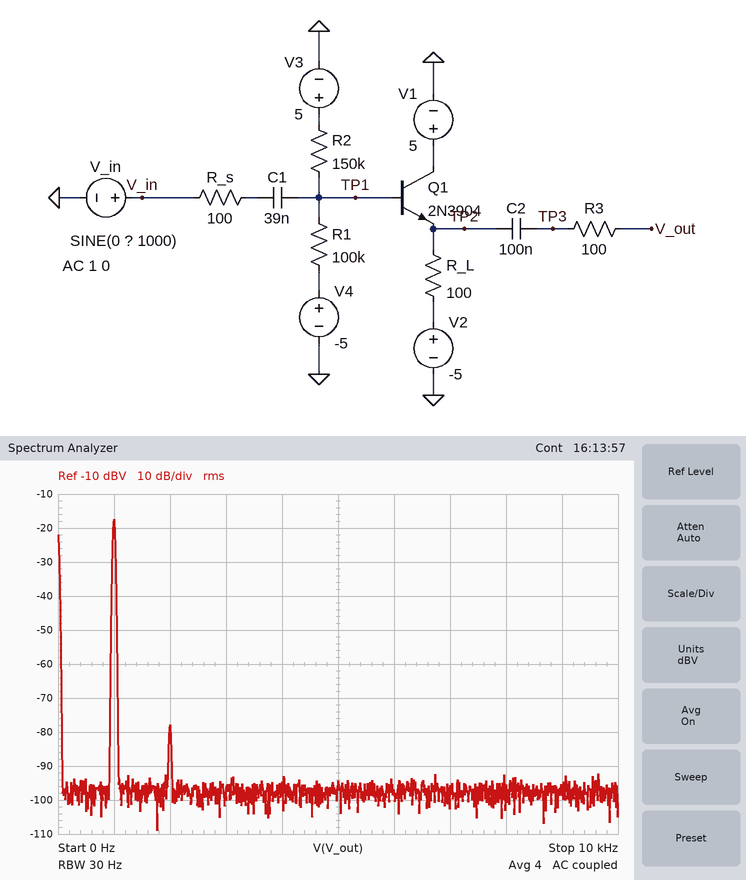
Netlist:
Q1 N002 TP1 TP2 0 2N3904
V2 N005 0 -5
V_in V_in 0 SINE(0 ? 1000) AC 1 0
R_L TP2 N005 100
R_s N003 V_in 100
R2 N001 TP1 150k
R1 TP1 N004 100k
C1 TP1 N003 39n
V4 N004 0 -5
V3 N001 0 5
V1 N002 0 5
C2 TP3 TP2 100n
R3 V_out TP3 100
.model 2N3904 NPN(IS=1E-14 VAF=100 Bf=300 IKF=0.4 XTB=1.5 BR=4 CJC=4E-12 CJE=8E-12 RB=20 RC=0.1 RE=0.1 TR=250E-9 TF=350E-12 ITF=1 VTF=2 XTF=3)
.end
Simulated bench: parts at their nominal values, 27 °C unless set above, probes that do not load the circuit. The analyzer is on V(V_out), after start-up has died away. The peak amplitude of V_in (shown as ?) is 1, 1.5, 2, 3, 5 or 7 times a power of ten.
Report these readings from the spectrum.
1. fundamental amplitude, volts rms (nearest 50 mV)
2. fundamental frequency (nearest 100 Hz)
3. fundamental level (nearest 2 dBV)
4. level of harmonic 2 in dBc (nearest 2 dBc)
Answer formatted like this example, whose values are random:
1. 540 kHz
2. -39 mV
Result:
1. 150 mV
2. 1.0 kHz
3. -18 dBV
4. -60 dBc
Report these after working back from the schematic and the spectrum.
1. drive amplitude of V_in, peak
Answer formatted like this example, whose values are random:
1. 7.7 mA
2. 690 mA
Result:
1. 200 mV
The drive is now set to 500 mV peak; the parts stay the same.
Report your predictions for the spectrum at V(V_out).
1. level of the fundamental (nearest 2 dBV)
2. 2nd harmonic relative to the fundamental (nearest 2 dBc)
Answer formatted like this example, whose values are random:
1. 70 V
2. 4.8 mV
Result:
1. -10 dBV
2. -52 dBc
